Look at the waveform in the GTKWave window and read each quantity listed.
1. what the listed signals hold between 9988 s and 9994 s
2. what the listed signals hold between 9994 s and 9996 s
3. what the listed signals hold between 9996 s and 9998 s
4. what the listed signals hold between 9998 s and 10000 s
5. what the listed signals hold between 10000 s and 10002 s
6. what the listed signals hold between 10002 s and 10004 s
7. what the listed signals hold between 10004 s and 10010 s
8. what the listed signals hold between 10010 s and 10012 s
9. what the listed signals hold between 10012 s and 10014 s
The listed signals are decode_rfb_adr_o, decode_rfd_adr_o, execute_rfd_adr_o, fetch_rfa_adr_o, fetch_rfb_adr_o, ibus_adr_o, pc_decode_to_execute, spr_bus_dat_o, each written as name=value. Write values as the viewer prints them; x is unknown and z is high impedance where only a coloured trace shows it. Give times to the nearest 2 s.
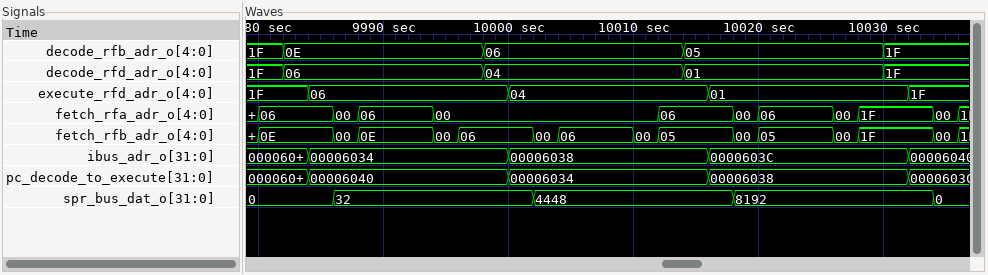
decode_rfb_adr_o=0E, decode_rfd_adr_o=06, execute_rfd_adr_o=06, fetch_rfa_adr_o=06, fetch_rfb_adr_o=0E, ibus_adr_o=00006034, pc_decode_to_execute=00006040, spr_bus_dat_o=32
decode_rfb_adr_o=0E, decode_rfd_adr_o=06, execute_rfd_adr_o=06, fetch_rfa_adr_o=00, fetch_rfb_adr_o=00, ibus_adr_o=00006034, pc_decode_to_execute=00006040, spr_bus_dat_o=32
decode_rfb_adr_o=0E, decode_rfd_adr_o=06, execute_rfd_adr_o=06, fetch_rfa_adr_o=00, fetch_rfb_adr_o=06, ibus_adr_o=00006034, pc_decode_to_execute=00006040, spr_bus_dat_o=32
decode_rfb_adr_o=06, decode_rfd_adr_o=04, execute_rfd_adr_o=06, fetch_rfa_adr_o=00, fetch_rfb_adr_o=06, ibus_adr_o=00006034, pc_decode_to_execute=00006040, spr_bus_dat_o=32
decode_rfb_adr_o=06, decode_rfd_adr_o=04, execute_rfd_adr_o=04, fetch_rfa_adr_o=00, fetch_rfb_adr_o=06, ibus_adr_o=00006038, pc_decode_to_execute=00006034, spr_bus_dat_o=32
decode_rfb_adr_o=06, decode_rfd_adr_o=04, execute_rfd_adr_o=04, fetch_rfa_adr_o=00, fetch_rfb_adr_o=00, ibus_adr_o=00006038, pc_decode_to_execute=00006034, spr_bus_dat_o=4448
decode_rfb_adr_o=06, decode_rfd_adr_o=04, execute_rfd_adr_o=04, fetch_rfa_adr_o=00, fetch_rfb_adr_o=06, ibus_adr_o=00006038, pc_decode_to_execute=00006034, spr_bus_dat_o=4448
decode_rfb_adr_o=06, decode_rfd_adr_o=04, execute_rfd_adr_o=04, fetch_rfa_adr_o=00, fetch_rfb_adr_o=00, ibus_adr_o=00006038, pc_decode_to_execute=00006034, spr_bus_dat_o=4448
decode_rfb_adr_o=06, decode_rfd_adr_o=04, execute_rfd_adr_o=04, fetch_rfa_adr_o=06, fetch_rfb_adr_o=05, ibus_adr_o=00006038, pc_decode_to_execute=00006034, spr_bus_dat_o=4448
